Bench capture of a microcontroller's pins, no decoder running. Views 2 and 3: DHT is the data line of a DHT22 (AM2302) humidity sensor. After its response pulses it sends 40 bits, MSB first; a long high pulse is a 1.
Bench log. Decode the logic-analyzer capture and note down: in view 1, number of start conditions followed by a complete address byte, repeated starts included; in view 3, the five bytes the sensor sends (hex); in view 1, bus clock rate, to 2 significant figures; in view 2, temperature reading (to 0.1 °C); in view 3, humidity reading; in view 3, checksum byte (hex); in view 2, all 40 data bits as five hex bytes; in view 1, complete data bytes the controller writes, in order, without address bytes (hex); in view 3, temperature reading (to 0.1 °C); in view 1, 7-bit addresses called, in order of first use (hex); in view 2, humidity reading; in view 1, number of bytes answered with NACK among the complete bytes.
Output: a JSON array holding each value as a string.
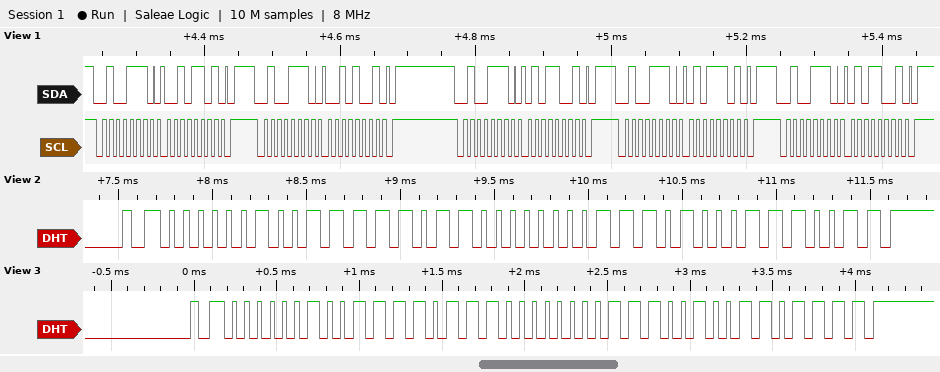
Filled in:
["5", "02 7B 80 72 6F", "100 kHz", "-11.6 °C", "63.5 %", "0x6F", "02 7D 80 74 73", "2D 29 59 5D 59", "-11.4 °C", "0x27", "63.7 %", "0"]
